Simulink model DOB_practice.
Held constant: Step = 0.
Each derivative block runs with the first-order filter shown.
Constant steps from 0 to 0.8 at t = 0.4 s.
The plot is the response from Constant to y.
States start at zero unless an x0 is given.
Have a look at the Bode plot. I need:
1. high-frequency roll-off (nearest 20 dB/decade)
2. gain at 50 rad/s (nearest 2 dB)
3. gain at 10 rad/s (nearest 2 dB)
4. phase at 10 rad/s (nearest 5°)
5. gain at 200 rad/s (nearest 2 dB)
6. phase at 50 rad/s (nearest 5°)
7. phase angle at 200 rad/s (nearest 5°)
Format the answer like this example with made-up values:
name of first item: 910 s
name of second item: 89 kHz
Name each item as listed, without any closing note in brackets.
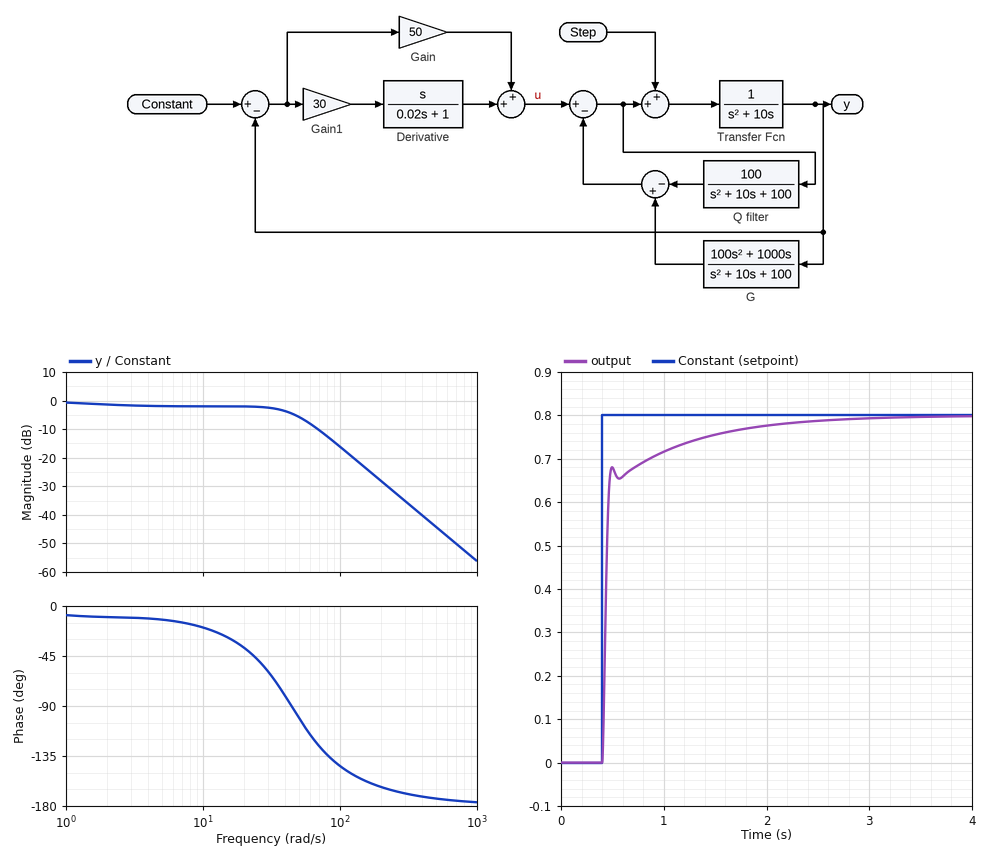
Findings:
high-frequency roll-off: -40 dB/decade
gain at 50 rad/s: -6 dB
gain at 10 rad/s: -2 dB
phase at 10 rad/s: -20°
gain at 200 rad/s: -28 dB
phase at 50 rad/s: -100°
phase angle at 200 rad/s: -165°
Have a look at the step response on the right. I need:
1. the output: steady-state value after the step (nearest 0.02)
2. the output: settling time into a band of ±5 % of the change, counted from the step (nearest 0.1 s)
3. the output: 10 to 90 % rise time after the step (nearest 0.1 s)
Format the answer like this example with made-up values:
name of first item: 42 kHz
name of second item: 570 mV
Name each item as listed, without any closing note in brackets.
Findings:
the output: steady-state value after the step: 0.80
the output: settling time into a band of ±5 % of the change, counted from the step: 1.2 s
the output: 10 to 90 % rise time after the step: 0.6 s
